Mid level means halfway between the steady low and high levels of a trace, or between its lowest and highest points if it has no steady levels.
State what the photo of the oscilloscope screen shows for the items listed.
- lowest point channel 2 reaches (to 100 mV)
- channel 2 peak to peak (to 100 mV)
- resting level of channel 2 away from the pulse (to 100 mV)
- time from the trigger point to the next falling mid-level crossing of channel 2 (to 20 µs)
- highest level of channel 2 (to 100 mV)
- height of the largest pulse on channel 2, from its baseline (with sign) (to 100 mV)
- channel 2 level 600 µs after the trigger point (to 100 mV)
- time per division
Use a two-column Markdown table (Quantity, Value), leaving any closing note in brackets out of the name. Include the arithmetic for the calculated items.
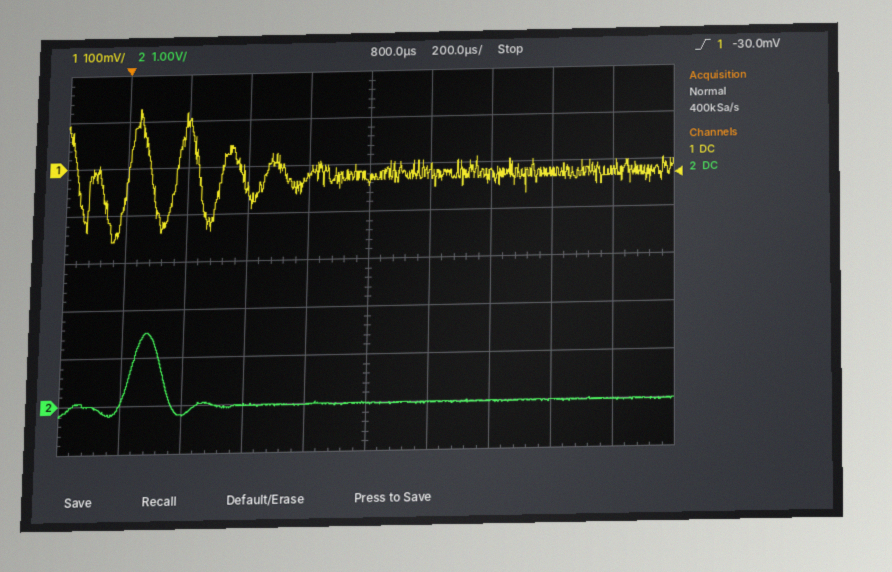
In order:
| Quantity | Value |
|---|---|
| lowest point channel 2 reaches | -200 mV |
| channel 2 peak to peak | 1.5 V − (-200 mV) = 1.7 V |
| resting level of channel 2 away from the pulse | 0.0 V |
| time from the trigger point to the next falling mid-level crossing of channel 2 | 140 µs |
| highest level of channel 2 | 1.5 V |
| height of the largest pulse on channel 2, from its baseline (with sign) | 1.5 V − (0.0 V) = +1.5 V |
| channel 2 level 600 µs after the trigger point | 0.0 V |
| time per division | 200 µs |
